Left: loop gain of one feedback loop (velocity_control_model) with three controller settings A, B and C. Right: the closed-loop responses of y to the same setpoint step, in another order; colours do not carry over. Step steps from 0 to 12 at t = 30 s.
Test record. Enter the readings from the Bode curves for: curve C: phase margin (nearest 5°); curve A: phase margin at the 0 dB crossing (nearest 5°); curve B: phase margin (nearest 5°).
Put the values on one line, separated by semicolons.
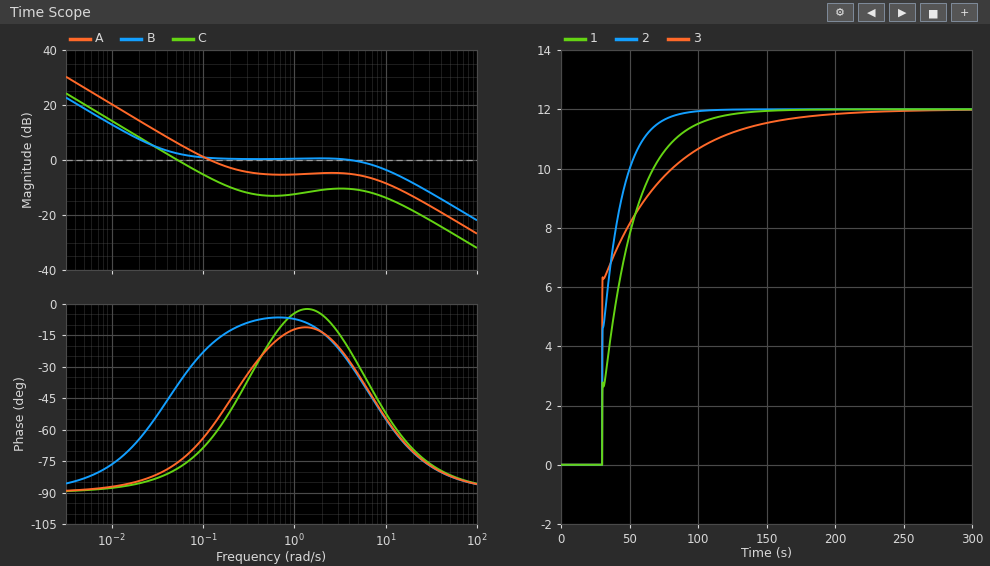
100°; 120°; 150°
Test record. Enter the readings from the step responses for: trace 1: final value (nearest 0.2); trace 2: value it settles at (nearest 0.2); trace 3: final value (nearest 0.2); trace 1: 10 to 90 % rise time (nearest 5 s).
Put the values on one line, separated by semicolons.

12.0; 12.0; 12.0; 50 s
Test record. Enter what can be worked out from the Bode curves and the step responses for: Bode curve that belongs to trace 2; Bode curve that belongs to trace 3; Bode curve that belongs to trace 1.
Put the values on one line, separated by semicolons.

A; B; C
